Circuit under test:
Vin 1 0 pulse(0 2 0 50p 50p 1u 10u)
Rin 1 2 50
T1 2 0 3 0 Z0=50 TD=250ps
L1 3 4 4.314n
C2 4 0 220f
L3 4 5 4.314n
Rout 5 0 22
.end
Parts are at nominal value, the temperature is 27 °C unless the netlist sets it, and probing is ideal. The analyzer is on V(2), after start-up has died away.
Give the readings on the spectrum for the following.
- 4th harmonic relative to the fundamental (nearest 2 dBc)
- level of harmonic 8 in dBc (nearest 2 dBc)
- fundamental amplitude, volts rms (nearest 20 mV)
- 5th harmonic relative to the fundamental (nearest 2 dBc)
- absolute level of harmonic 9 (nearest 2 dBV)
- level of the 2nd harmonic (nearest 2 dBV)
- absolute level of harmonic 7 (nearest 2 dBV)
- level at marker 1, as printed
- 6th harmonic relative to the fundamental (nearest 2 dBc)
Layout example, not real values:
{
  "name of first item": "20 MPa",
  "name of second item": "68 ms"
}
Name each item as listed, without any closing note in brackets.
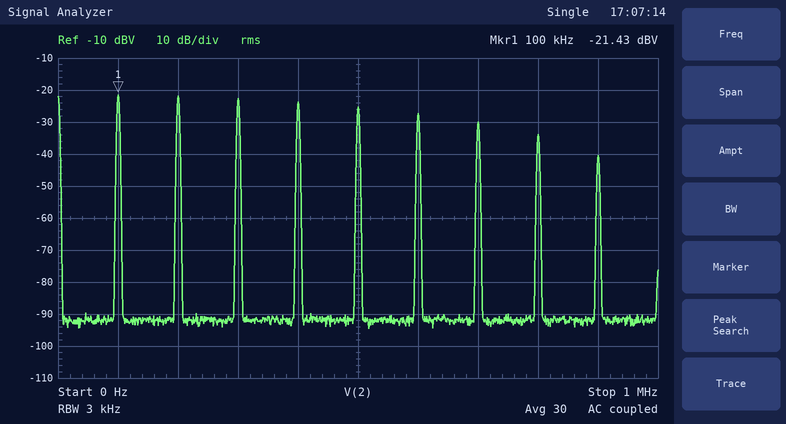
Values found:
{
  "4th harmonic relative to the fundamental": "-2 dBc",
  "level of harmonic 8 in dBc": "-12 dBc",
  "fundamental amplitude, volts rms": "80 mV",
  "5th harmonic relative to the fundamental": "-4 dBc",
  "absolute level of harmonic 9": "-40 dBV",
  "level of the 2nd harmonic": "-22 dBV",
  "absolute level of harmonic 7": "-30 dBV",
  "level at marker 1, as printed": "-21.43 dBV",
  "6th harmonic relative to the fundamental": "-6 dBc"
}
